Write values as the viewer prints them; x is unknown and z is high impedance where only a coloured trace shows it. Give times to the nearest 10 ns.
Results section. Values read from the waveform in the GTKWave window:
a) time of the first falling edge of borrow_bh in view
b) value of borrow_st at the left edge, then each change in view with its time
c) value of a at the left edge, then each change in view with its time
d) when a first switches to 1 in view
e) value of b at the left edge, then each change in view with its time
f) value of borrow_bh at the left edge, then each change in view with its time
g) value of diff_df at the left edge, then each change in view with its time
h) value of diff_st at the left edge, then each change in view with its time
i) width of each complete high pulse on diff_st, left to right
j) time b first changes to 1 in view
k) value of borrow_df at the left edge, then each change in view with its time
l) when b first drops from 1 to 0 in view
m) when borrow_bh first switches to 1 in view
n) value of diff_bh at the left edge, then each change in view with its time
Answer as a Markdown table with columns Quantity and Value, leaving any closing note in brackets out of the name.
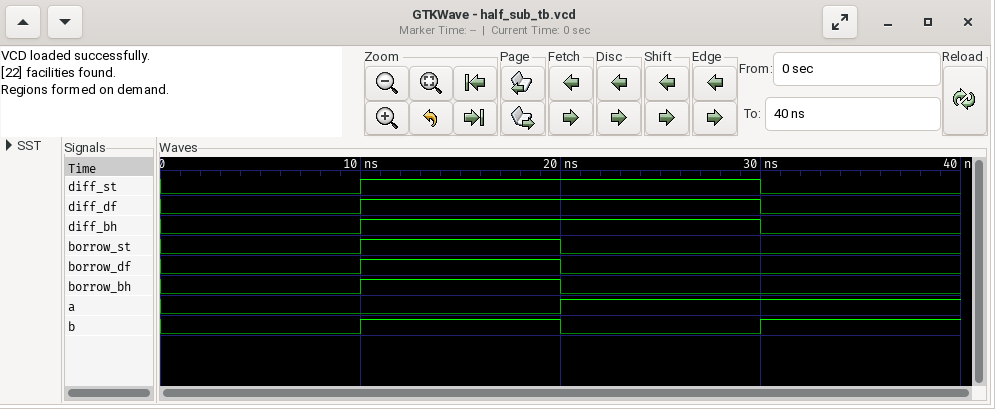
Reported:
| Quantity | Value |
|---|---|
| time of the first falling edge of borrow_bh in view | 20 ns |
| value of borrow_st at the left edge, then each change in view with its time | 0, 1 at 10 ns, 0 at 20 ns |
| value of a at the left edge, then each change in view with its time | 0, 1 at 20 ns |
| when a first switches to 1 in view | 20 ns |
| value of b at the left edge, then each change in view with its time | 0, 1 at 10 ns, 0 at 20 ns, 1 at 30 ns |
| value of borrow_bh at the left edge, then each change in view with its time | 0, 1 at 10 ns, 0 at 20 ns |
| value of diff_df at the left edge, then each change in view with its time | 0, 1 at 10 ns, 0 at 30 ns |
| value of diff_st at the left edge, then each change in view with its time | 0, 1 at 10 ns, 0 at 30 ns |
| width of each complete high pulse on diff_st, left to right | 20 ns |
| time b first changes to 1 in view | 10 ns |
| value of borrow_df at the left edge, then each change in view with its time | 0, 1 at 10 ns, 0 at 20 ns |
| when b first drops from 1 to 0 in view | 20 ns |
| when borrow_bh first switches to 1 in view | 10 ns |
| value of diff_bh at the left edge, then each change in view with its time | 0, 1 at 10 ns, 0 at 30 ns |
